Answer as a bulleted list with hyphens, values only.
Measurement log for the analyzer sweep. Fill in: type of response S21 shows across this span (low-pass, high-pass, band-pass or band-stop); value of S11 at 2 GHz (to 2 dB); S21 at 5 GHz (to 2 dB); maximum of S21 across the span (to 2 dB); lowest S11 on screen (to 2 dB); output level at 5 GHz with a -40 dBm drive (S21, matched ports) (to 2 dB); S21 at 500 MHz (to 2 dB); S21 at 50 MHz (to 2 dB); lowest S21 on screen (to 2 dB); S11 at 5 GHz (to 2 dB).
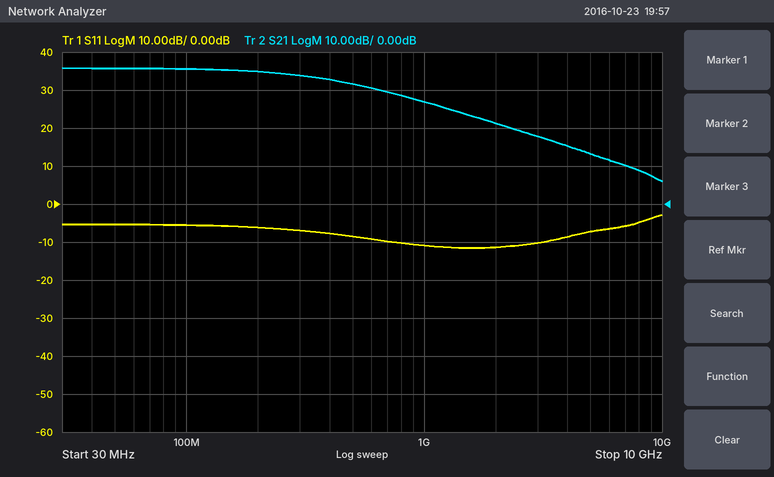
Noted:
- low-pass
- -12 dB
- 14 dB
- 36 dB
- -12 dB
- -26 dBm
- 32 dB
- 36 dB
- 6 dB
- -8 dB
